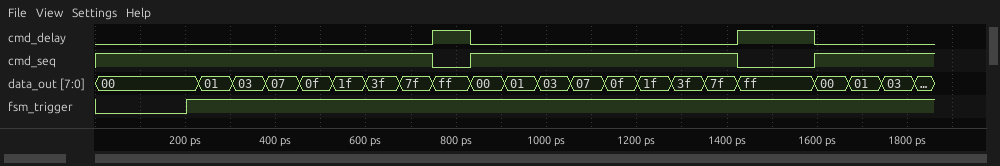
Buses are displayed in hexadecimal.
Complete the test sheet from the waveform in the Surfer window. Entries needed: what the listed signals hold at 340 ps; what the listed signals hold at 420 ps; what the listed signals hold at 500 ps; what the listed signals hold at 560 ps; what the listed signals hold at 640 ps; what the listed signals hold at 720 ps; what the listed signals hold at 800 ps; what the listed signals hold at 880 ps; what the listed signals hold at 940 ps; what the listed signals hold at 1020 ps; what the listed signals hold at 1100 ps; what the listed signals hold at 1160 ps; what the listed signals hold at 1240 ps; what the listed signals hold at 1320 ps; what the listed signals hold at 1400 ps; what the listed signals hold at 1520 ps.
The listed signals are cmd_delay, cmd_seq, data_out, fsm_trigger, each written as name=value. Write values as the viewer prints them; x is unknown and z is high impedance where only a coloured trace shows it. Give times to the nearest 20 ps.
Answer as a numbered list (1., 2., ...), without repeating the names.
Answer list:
1. cmd_delay=0, cmd_seq=1, data_out=03, fsm_trigger=1
2. cmd_delay=0, cmd_seq=1, data_out=07, fsm_trigger=1
3. cmd_delay=0, cmd_seq=1, data_out=0f, fsm_trigger=1
4. cmd_delay=0, cmd_seq=1, data_out=1f, fsm_trigger=1
5. cmd_delay=0, cmd_seq=1, data_out=3f, fsm_trigger=1
6. cmd_delay=0, cmd_seq=1, data_out=7f, fsm_trigger=1
7. cmd_delay=1, cmd_seq=0, data_out=ff, fsm_trigger=1
8. cmd_delay=0, cmd_seq=1, data_out=00, fsm_trigger=1
9. cmd_delay=0, cmd_seq=1, data_out=01, fsm_trigger=1
10. cmd_delay=0, cmd_seq=1, data_out=03, fsm_trigger=1
11. cmd_delay=0, cmd_seq=1, data_out=07, fsm_trigger=1
12. cmd_delay=0, cmd_seq=1, data_out=0f, fsm_trigger=1
13. cmd_delay=0, cmd_seq=1, data_out=1f, fsm_trigger=1
14. cmd_delay=0, cmd_seq=1, data_out=3f, fsm_trigger=1
15. cmd_delay=0, cmd_seq=1, data_out=7f, fsm_trigger=1
16. cmd_delay=1, cmd_seq=0, data_out=ff, fsm_trigger=1
